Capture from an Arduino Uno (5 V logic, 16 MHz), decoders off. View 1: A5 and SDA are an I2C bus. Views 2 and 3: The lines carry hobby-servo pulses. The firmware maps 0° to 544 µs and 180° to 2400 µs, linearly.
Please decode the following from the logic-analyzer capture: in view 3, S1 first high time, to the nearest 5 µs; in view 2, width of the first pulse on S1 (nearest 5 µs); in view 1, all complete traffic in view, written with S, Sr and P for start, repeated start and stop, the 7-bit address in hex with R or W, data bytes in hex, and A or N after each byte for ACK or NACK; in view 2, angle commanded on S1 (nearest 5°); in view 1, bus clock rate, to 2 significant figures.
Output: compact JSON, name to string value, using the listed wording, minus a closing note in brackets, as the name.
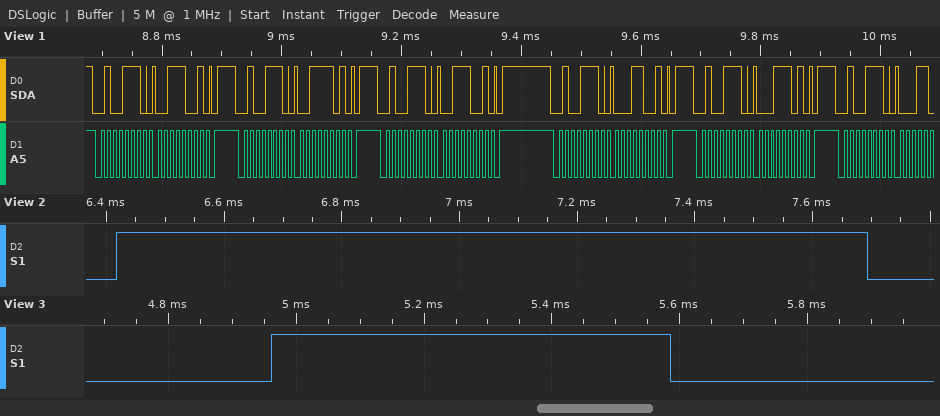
{"in view 3, S1 first high time, to the nearest 5 µs": "625 µs", "in view 2, width of the first pulse on S1": "1275 µs", "in view 1, all complete traffic in view, written with S, Sr and P for start, repeated start and stop, the 7-bit address in hex with R or W, data bytes in hex, and A or N after each byte for ACK or NACK": "S 27W A 39 A P S 27W A 3D A P S 27W A 39 A P S 27W A 19 A P S 27W A 1D A P S 27W A", "in view 2, angle commanded on S1": "70°", "in view 1, bus clock rate, to 2 significant figures": "100 kHz"}
